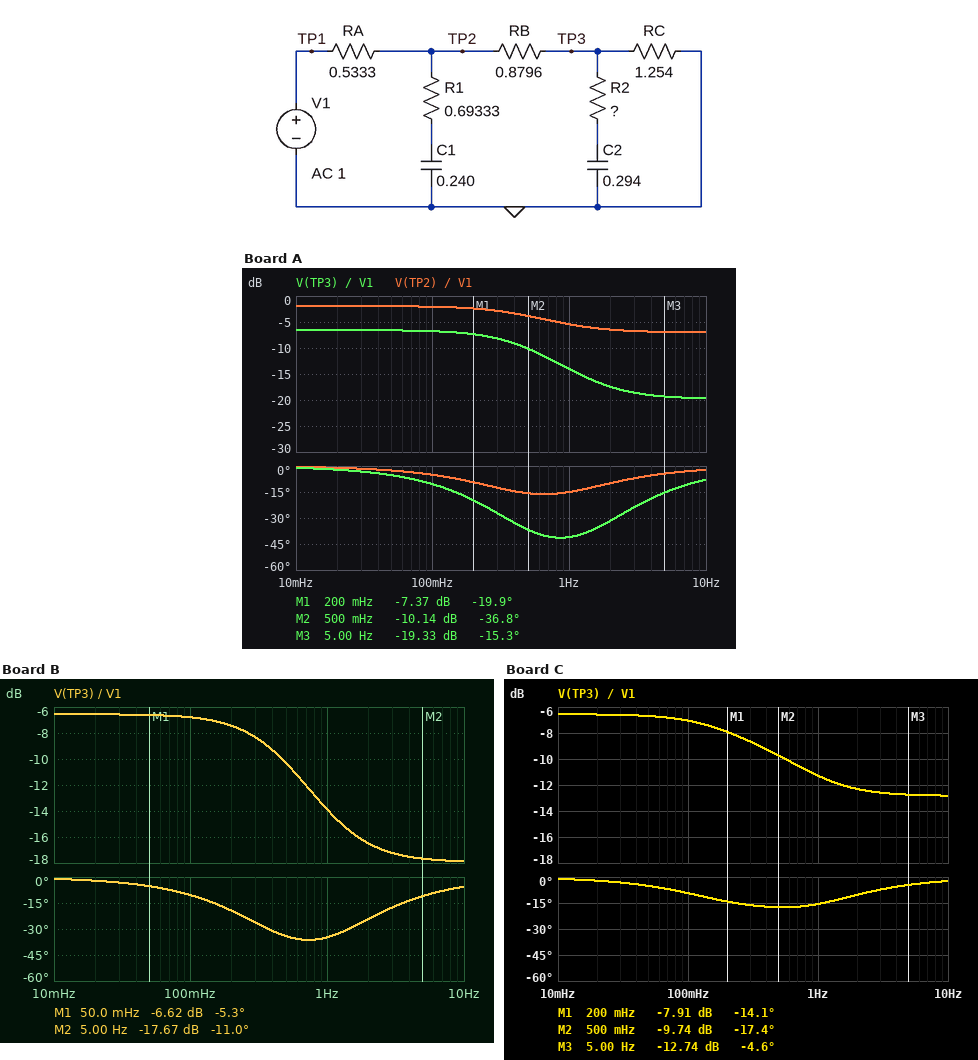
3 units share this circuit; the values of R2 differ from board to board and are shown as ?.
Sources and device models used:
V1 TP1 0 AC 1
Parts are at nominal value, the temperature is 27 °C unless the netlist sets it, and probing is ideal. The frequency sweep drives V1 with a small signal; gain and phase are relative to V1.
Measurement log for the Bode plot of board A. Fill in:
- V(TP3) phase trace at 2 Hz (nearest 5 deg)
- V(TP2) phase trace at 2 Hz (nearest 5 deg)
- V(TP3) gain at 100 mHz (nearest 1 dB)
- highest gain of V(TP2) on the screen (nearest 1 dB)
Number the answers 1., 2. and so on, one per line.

1. -30 deg
2. -10 deg
3. -7 dB
4. -2 dB
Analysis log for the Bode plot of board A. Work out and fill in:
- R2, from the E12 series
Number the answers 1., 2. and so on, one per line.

1. 0.33 Ω
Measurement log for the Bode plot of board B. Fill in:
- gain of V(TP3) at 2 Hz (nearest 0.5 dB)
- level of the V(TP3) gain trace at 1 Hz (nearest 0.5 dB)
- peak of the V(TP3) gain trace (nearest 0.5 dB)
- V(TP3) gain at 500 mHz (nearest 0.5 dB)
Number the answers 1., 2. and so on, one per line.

1. -16.5 dB
2. -14.0 dB
3. -6.5 dB
4. -10.5 dB
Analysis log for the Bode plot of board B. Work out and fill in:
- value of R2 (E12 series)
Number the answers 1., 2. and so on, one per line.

1. 0.47 Ω
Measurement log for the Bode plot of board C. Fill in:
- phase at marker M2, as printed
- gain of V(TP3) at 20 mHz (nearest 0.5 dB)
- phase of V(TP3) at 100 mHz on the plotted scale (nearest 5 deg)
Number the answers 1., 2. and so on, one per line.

1. -17.4 deg
2. -6.5 dB
3. -10 deg
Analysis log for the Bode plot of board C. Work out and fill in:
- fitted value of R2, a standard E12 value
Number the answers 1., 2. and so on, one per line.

1. 2.2 Ω
